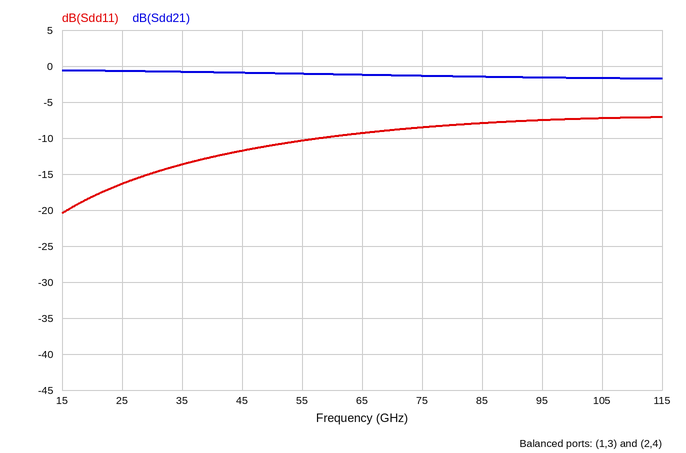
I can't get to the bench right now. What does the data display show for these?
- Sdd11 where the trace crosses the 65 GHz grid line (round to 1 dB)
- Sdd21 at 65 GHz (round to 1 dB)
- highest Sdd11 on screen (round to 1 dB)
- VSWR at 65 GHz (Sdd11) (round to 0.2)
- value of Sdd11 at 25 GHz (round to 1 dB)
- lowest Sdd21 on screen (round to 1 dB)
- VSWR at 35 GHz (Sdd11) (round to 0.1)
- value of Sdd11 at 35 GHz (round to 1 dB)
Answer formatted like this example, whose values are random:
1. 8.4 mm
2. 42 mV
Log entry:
1. -9 dB
2. -1 dB
3. -7 dB
4. 2.0
5. -16 dB
6. -2 dB
7. 1.5
8. -14 dB
